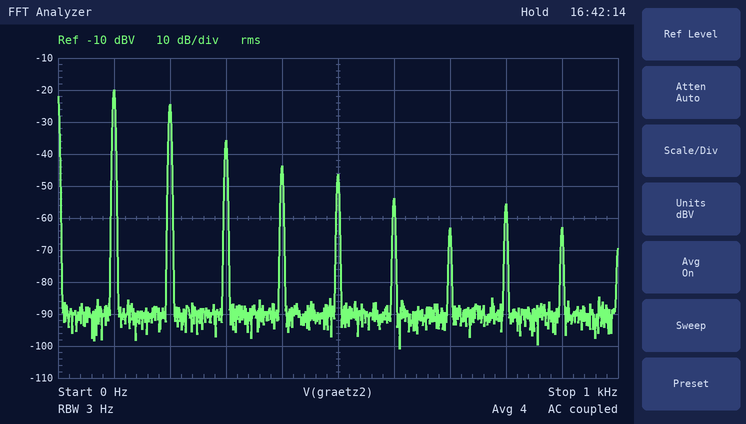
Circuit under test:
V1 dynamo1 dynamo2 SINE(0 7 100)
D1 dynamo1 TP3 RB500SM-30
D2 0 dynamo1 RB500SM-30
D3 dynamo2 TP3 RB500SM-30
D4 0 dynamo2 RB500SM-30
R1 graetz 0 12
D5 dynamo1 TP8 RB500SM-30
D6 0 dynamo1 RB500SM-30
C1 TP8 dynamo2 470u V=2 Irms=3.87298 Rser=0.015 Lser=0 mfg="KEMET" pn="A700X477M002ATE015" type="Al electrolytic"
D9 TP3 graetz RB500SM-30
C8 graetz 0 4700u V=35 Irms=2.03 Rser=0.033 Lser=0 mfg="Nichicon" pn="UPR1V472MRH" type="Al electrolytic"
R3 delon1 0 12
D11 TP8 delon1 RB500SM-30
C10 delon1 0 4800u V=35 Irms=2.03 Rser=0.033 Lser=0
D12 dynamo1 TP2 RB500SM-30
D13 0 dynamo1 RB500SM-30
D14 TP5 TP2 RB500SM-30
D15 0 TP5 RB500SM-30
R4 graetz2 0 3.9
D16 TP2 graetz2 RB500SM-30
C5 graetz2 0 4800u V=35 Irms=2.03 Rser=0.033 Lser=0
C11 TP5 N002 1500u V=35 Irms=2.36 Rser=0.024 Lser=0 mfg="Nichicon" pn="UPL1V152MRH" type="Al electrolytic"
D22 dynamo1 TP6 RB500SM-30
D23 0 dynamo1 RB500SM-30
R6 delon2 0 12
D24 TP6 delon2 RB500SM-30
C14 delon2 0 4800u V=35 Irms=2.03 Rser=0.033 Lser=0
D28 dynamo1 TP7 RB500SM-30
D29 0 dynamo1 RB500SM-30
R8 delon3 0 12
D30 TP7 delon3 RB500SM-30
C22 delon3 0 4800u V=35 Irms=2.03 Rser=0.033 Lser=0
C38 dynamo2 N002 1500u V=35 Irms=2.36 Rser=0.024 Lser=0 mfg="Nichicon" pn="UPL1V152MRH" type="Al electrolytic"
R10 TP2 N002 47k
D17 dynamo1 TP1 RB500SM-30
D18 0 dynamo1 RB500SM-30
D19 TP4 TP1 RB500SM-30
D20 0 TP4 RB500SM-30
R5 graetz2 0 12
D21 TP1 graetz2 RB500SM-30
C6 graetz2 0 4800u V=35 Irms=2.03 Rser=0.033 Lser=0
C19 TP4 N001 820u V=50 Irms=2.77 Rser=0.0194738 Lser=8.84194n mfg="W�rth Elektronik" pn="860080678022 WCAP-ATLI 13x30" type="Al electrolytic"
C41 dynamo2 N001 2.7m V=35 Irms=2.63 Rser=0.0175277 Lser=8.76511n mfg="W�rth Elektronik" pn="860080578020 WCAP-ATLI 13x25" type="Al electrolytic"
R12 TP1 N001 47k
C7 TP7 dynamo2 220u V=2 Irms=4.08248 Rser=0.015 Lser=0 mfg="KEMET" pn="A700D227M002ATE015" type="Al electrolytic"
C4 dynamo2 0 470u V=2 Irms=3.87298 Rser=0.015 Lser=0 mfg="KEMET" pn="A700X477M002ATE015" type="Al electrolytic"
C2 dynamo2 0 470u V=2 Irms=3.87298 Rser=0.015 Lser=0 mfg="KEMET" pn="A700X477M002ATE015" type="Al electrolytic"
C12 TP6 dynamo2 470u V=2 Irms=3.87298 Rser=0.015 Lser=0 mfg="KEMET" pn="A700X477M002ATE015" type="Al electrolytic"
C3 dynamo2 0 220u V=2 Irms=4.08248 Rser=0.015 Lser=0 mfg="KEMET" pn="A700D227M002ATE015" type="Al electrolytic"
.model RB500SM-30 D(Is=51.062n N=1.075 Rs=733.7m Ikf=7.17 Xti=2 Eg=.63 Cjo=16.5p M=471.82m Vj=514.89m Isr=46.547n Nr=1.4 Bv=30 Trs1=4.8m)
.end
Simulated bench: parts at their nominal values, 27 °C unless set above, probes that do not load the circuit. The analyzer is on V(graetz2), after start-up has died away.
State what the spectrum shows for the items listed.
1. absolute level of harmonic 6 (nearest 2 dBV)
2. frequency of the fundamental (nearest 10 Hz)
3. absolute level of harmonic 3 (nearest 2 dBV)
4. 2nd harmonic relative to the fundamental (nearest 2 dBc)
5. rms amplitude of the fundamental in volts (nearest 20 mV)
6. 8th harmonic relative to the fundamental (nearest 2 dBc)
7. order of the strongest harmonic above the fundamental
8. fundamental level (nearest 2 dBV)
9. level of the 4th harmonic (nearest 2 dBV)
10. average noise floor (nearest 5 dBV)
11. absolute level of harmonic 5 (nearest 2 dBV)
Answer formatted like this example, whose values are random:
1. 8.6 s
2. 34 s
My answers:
1. -54 dBV
2. 100 Hz
3. -36 dBV
4. -4 dBc
5. 100 mV
6. -36 dBc
7. 2
8. -20 dBV
9. -44 dBV
10. -90 dBV
11. -46 dBV
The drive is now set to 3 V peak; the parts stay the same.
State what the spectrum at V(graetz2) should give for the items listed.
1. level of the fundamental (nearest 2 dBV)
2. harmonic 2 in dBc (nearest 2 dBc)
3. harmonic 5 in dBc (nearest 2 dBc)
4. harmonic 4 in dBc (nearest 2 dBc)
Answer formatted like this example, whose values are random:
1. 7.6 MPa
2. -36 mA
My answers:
1. -28 dBV
2. -8 dBc
3. -30 dBc
4. -26 dBc
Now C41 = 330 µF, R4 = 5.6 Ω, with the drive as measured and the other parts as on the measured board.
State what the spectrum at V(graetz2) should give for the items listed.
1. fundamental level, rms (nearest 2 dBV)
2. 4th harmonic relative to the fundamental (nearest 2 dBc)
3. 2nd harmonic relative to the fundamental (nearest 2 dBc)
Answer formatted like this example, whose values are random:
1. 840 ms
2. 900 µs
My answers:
1. -20 dBV
2. -28 dBc
3. -6 dBc
